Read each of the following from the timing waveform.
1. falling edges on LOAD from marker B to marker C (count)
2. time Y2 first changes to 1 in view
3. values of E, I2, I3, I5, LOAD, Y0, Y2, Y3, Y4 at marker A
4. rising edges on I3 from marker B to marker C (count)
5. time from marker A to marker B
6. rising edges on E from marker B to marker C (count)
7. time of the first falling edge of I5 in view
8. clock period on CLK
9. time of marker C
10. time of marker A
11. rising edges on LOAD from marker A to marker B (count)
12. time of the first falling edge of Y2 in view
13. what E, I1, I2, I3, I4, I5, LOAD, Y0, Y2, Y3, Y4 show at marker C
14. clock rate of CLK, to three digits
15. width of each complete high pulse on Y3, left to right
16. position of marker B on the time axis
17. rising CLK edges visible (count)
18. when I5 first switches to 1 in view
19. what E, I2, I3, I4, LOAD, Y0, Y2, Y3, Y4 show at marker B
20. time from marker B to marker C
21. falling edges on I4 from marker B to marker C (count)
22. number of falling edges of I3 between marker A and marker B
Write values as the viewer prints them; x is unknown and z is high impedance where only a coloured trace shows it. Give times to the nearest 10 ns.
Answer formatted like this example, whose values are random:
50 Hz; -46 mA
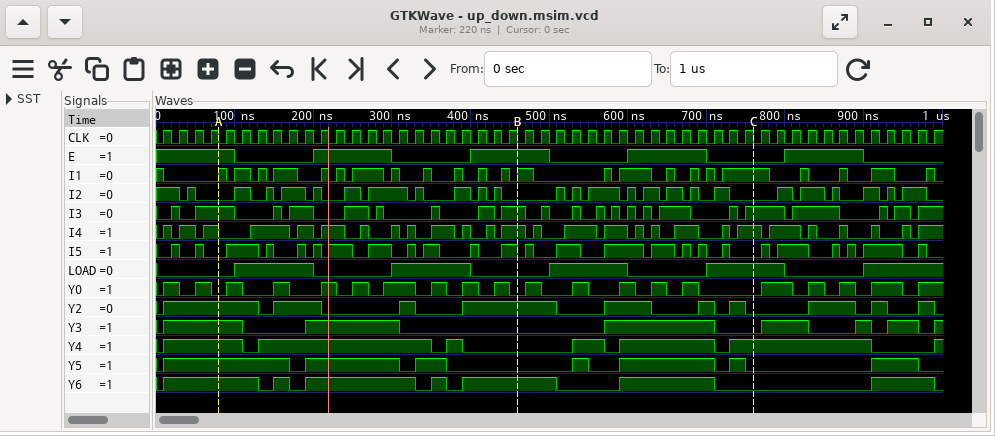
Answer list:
1; 10 ns; E=1, I2=0, I3=1, I5=0, LOAD=0, Y0=0, Y2=1, Y3=1, Y4=1; 9; 380 ns; 1; 30 ns; 20 ns; 760 ns; 80 ns; 2; 130 ns; E=0, I1=1, I2=0, I3=1, I4=1, I5=0, LOAD=1, Y0=0, Y2=0, Y3=0, Y4=1; 50.0 MHz; 100 ns, 120 ns, 140 ns, 60 ns, 20 ns, 40 ns; 460 ns; 50; 20 ns; E=1, I2=0, I3=1, I4=1, LOAD=0, Y0=0, Y2=1, Y3=0, Y4=0; 300 ns; 8; 7
